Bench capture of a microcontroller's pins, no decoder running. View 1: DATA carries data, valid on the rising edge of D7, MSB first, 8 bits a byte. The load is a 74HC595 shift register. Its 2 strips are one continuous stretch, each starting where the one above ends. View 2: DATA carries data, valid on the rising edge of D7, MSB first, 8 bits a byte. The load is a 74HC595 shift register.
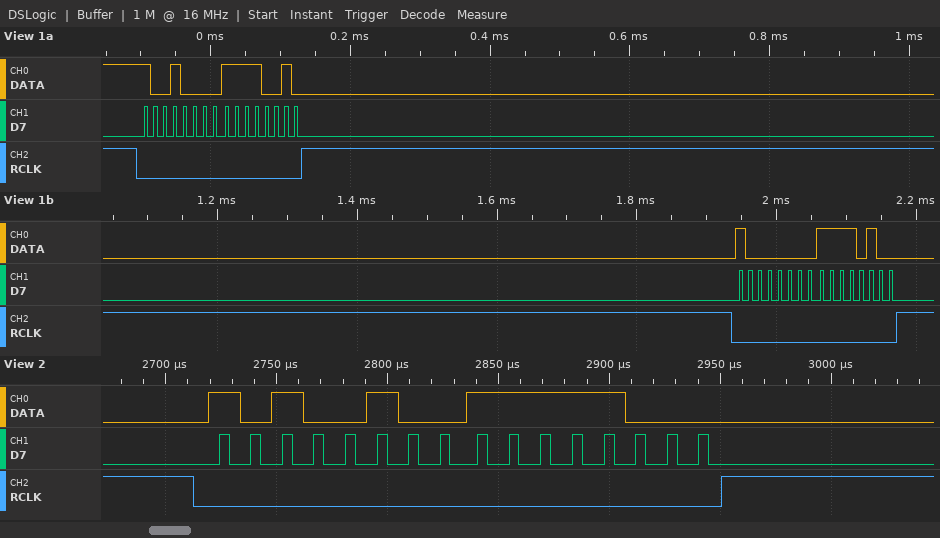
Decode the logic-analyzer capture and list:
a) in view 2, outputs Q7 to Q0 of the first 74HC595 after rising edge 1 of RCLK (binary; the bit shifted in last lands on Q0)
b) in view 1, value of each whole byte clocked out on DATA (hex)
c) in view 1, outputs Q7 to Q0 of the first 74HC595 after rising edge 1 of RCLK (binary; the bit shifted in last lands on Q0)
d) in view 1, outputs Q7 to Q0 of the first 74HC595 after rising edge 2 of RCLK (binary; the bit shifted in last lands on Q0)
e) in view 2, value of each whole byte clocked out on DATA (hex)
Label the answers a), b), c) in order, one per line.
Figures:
a) 11111000
b) 90 F2 80 F4
c) 11110010
d) 11110100
e) A4 F8
